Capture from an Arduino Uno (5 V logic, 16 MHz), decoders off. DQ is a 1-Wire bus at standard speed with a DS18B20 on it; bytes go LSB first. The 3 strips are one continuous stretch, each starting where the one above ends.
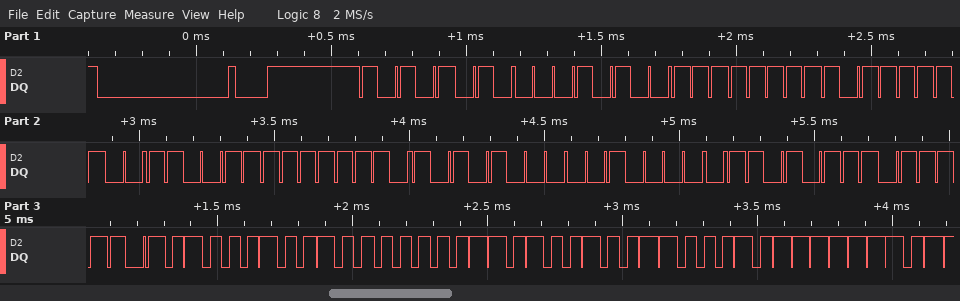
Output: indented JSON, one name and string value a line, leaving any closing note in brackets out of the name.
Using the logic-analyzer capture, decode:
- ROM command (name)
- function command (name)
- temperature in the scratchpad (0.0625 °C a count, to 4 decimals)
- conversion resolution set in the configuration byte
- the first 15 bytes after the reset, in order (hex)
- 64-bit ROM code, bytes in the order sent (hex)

{
  "ROM command": "Match ROM",
  "function command": "Read Scratchpad",
  "temperature in the scratchpad": "18.1250 °C",
  "conversion resolution set in the configuration byte": "12 bits",
  "the first 15 bytes after the reset, in order": "55 28 FF FD CC 7F 15 04 EB BE 22 01 4B 46 7F",
  "64-bit ROM code, bytes in the order sent": "28 FF FD CC 7F 15 04 EB"
}
